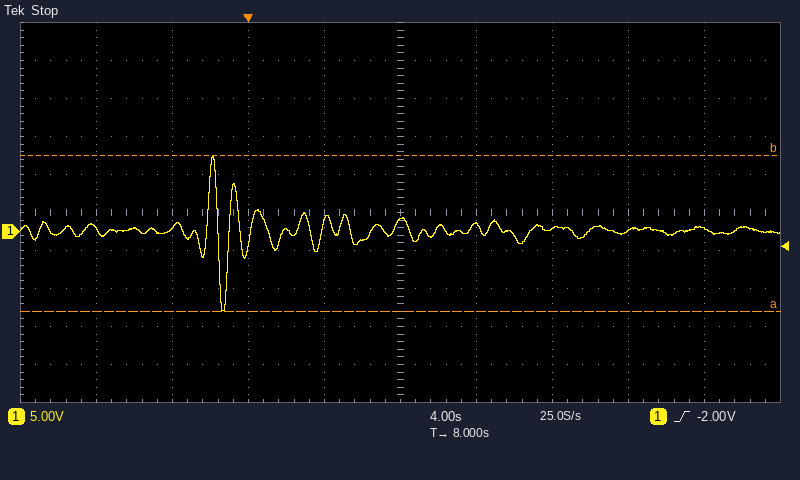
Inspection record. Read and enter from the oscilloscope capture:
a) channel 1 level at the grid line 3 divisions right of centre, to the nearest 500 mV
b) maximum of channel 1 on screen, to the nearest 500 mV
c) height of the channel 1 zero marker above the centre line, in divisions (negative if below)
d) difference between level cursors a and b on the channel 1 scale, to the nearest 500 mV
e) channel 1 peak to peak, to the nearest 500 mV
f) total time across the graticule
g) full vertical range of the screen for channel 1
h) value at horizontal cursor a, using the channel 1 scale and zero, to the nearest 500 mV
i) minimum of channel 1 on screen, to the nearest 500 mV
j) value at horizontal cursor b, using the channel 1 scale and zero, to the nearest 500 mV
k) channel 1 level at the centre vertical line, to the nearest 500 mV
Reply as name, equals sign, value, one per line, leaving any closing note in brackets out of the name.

channel 1 level at the grid line 3 divisions right of centre, to the nearest 500 mV = 0.0 V
maximum of channel 1 on screen, to the nearest 500 mV = 10.0 V
height of the channel 1 zero marker above the centre line, in divisions = -0.5 div
difference between level cursors a and b on the channel 1 scale, to the nearest 500 mV = 20.5 V
channel 1 peak to peak, to the nearest 500 mV = 20.5 V
total time across the graticule = 40 s
full vertical range of the screen for channel 1 = 50 V
value at horizontal cursor a, using the channel 1 scale and zero, to the nearest 500 mV = -10.5 V
minimum of channel 1 on screen, to the nearest 500 mV = -10.5 V
value at horizontal cursor b, using the channel 1 scale and zero, to the nearest 500 mV = 10.0 V
channel 1 level at the centre vertical line, to the nearest 500 mV = 1.5 V
